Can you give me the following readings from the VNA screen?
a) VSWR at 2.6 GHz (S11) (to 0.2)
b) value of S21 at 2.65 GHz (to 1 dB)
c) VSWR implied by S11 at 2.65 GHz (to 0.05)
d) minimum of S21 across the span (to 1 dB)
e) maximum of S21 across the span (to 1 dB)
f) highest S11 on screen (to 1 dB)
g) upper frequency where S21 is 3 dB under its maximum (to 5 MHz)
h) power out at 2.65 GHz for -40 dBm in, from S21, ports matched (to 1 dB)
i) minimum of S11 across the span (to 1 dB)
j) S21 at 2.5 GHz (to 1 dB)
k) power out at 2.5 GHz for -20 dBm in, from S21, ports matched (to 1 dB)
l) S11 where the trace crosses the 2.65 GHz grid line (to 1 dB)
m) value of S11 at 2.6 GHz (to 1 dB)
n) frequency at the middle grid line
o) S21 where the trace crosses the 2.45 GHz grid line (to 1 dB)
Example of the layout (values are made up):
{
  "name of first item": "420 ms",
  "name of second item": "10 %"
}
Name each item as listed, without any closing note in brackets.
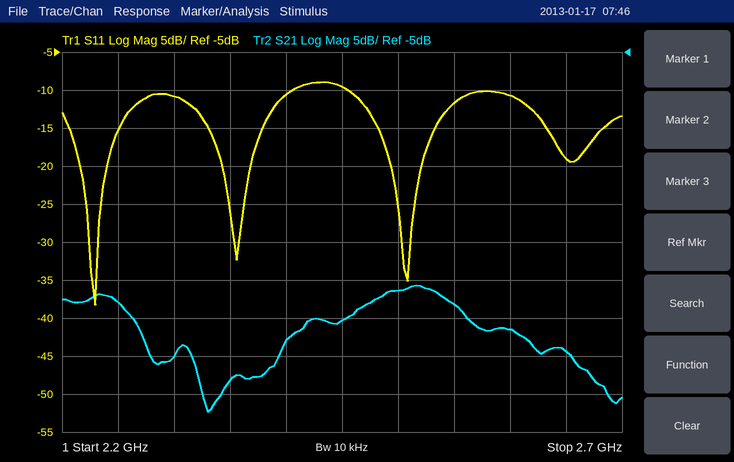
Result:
{
  "VSWR at 2.6 GHz (S11)": "1.8",
  "value of S21 at 2.65 GHz": "-44 dB",
  "VSWR implied by S11 at 2.65 GHz": "1.25",
  "minimum of S21 across the span": "-52 dB",
  "maximum of S21 across the span": "-36 dB",
  "highest S11 on screen": "-9 dB",
  "upper frequency where S21 is 3 dB under its maximum": "2.555 GHz",
  "power out at 2.65 GHz for -40 dBm in, from S21, ports matched": "-84 dBm",
  "minimum of S11 across the span": "-38 dB",
  "S21 at 2.5 GHz": "-36 dB",
  "power out at 2.5 GHz for -20 dBm in, from S21, ports matched": "-56 dBm",
  "S11 where the trace crosses the 2.65 GHz grid line": "-19 dB",
  "value of S11 at 2.6 GHz": "-11 dB",
  "frequency at the middle grid line": "2.45 GHz",
  "S21 where the trace crosses the 2.45 GHz grid line": "-40 dB"
}
